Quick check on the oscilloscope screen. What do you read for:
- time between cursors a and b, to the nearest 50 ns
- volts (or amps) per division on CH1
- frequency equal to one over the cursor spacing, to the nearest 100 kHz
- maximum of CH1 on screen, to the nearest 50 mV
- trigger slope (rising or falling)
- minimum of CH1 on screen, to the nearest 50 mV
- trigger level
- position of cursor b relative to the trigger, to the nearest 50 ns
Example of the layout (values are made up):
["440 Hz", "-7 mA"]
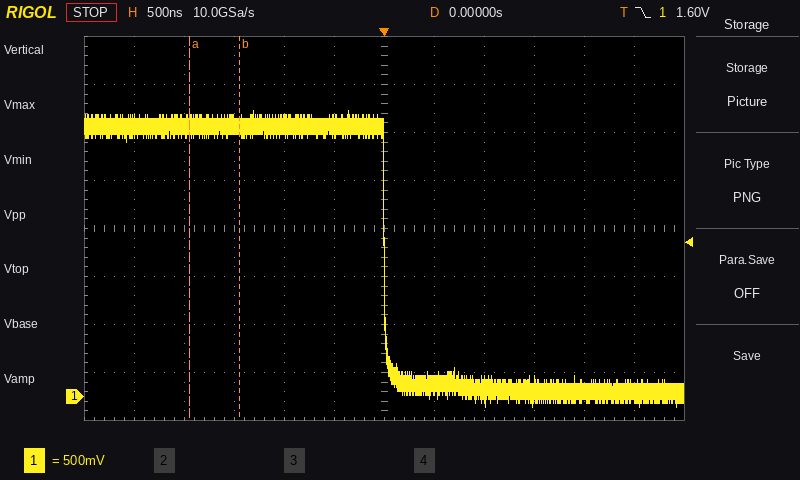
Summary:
["500 ns", "500 mV", "2.0 MHz", "3.00 V", "falling", "-100 mV", "1.60 V", "-1.45 µs"]
